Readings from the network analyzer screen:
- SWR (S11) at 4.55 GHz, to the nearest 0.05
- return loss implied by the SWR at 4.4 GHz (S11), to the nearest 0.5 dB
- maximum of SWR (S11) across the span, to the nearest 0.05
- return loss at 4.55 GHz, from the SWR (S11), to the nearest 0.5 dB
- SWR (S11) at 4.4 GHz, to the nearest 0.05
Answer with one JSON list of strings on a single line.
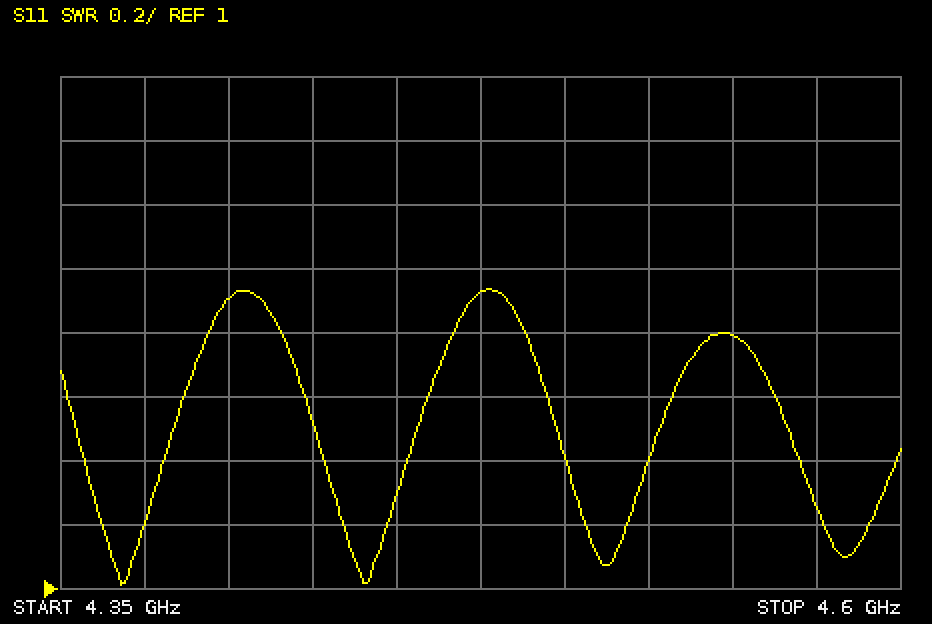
["1.80", "10.0 dB", "1.95", "11.0 dB", "1.90"]
